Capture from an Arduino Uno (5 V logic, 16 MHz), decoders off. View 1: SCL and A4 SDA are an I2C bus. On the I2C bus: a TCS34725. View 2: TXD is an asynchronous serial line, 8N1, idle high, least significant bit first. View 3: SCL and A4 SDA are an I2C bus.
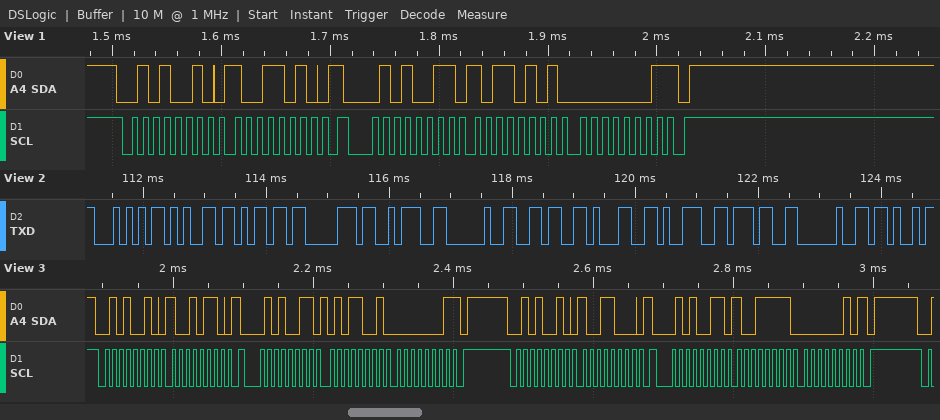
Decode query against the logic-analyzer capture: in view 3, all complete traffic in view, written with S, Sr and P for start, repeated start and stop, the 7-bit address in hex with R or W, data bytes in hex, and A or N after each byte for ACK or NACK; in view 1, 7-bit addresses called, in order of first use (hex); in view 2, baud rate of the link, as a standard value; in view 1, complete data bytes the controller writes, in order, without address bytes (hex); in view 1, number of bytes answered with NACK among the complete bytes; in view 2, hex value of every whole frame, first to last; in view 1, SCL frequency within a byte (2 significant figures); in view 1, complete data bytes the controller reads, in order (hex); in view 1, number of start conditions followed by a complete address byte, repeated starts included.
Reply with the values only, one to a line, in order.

S 29W A 96 A Sr 29R A 59 A 01 N P S 29W A 98 A Sr 29R A 9F A 02 N P
0x29
9600 baud
9A
1
54 65 6D 70 3A 20 36 31 39 37 20 4B
100 kHz
B5 01
2
